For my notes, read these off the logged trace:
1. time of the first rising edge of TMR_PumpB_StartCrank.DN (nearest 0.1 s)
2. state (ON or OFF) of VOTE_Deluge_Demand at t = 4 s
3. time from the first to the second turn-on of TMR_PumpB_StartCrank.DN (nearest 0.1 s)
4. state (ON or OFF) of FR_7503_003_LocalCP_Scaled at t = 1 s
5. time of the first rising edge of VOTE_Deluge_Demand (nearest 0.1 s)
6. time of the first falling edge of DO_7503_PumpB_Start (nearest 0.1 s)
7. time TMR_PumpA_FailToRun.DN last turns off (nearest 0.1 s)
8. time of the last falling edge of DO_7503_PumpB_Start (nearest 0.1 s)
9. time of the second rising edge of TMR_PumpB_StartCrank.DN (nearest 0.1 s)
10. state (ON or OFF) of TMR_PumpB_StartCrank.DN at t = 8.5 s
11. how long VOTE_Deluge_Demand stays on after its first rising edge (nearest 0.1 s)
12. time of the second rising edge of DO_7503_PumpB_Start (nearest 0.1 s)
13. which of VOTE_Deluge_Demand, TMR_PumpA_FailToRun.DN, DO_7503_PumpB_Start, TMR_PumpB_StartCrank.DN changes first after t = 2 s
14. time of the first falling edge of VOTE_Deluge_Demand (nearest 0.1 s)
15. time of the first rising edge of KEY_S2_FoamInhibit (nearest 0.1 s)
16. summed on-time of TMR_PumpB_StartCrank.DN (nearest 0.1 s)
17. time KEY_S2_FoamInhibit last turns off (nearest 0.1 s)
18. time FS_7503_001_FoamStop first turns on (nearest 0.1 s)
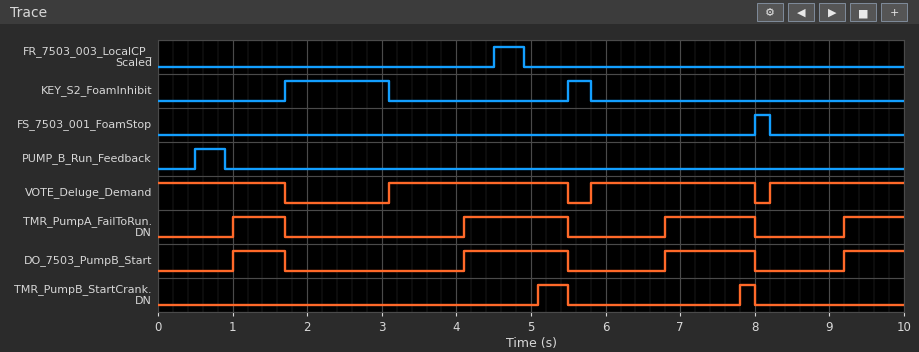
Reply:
5.1 s
ON
2.7 s
OFF
3.1 s
1.7 s
8.0 s
8.0 s
7.8 s
OFF
2.4 s
4.1 s
VOTE_Deluge_Demand
1.7 s
1.7 s
0.6 s
5.8 s
8.0 s
